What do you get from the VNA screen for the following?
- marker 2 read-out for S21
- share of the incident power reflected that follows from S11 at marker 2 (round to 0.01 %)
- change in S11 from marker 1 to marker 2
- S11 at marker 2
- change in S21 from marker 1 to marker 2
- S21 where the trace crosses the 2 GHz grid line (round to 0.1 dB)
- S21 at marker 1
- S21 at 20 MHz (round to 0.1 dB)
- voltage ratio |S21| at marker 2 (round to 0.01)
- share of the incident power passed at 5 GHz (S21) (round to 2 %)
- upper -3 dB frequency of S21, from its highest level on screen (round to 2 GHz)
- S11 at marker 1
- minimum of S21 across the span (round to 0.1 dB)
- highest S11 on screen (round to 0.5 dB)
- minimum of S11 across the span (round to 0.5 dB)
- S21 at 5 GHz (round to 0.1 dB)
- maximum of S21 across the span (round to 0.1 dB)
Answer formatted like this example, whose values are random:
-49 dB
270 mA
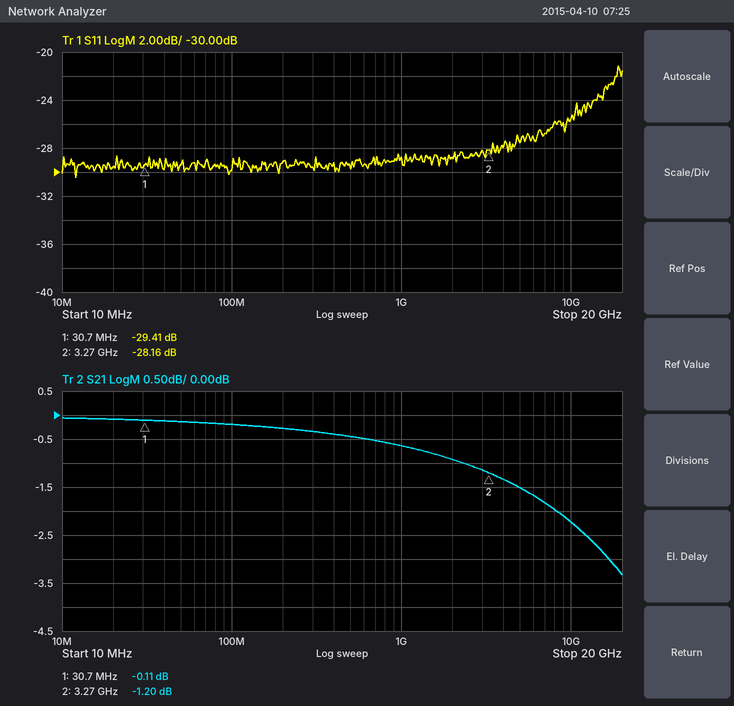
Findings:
-1.20 dB
0.15 %
1.25 dB
-28.16 dB
-1.09 dB
-0.9 dB
-0.11 dB
-0.1 dB
0.87
70 %
18 GHz
-29.41 dB
-3.3 dB
-21.0 dB
-30.5 dB
-1.5 dB
-0.1 dB
